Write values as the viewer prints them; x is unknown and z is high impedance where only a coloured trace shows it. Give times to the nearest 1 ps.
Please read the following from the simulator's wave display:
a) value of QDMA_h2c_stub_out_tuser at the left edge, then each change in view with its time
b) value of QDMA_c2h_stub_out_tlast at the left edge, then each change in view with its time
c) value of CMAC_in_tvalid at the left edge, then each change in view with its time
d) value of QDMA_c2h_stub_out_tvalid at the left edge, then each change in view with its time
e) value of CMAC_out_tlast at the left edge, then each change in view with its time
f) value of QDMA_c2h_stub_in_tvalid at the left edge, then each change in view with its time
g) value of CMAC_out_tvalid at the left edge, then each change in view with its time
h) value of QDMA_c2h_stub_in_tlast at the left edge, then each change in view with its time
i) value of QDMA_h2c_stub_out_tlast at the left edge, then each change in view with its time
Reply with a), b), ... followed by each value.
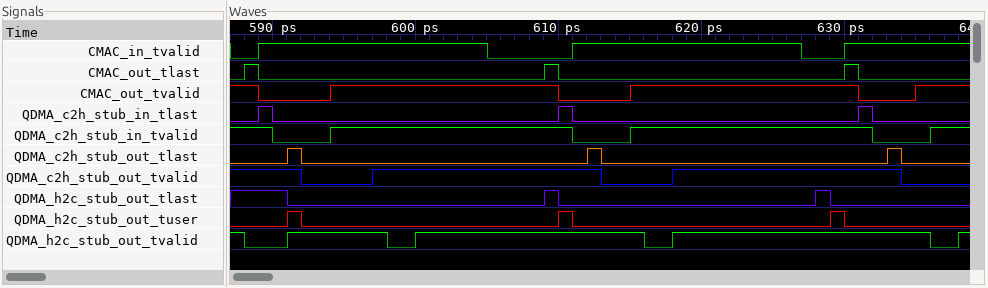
a) 0, 1 at 591 ps, 0 at 592 ps, 1 at 610 ps, 0 at 611 ps, 1 at 629 ps, 0 at 630 ps
b) 0, 1 at 591 ps, 0 at 592 ps, 1 at 612 ps, 0 at 613 ps, 1 at 633 ps, 0 at 634 ps
c) 0, 1 at 589 ps, 0 at 605 ps, 1 at 611 ps, 0 at 627 ps, 1 at 630 ps
d) 1, 0 at 592 ps, 1 at 597 ps, 0 at 613 ps, 1 at 618 ps, 0 at 634 ps
e) 0, 1 at 588 ps, 0 at 589 ps, 1 at 609 ps, 0 at 610 ps, 1 at 630 ps, 0 at 631 ps
f) 1, 0 at 590 ps, 1 at 594 ps, 0 at 611 ps, 1 at 615 ps, 0 at 632 ps, 1 at 636 ps
g) 1, 0 at 589 ps, 1 at 594 ps, 0 at 610 ps, 1 at 615 ps, 0 at 631 ps, 1 at 635 ps
h) 0, 1 at 589 ps, 0 at 590 ps, 1 at 610 ps, 0 at 611 ps, 1 at 631 ps, 0 at 632 ps
i) 1, 0 at 591 ps, 1 at 609 ps, 0 at 610 ps, 1 at 628 ps, 0 at 629 ps
